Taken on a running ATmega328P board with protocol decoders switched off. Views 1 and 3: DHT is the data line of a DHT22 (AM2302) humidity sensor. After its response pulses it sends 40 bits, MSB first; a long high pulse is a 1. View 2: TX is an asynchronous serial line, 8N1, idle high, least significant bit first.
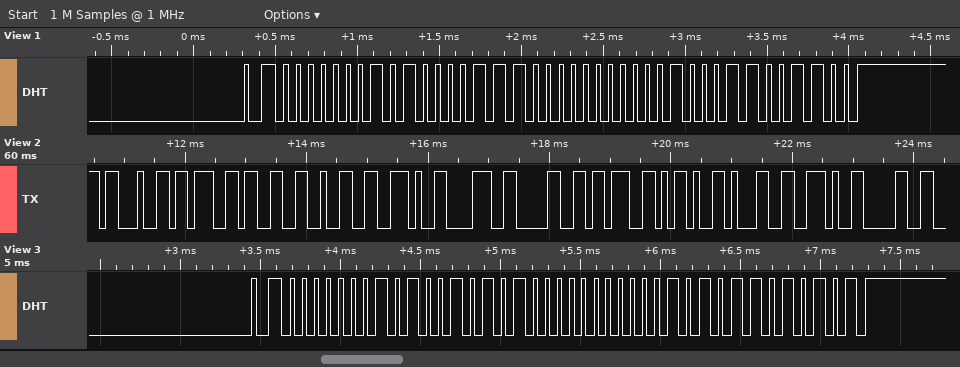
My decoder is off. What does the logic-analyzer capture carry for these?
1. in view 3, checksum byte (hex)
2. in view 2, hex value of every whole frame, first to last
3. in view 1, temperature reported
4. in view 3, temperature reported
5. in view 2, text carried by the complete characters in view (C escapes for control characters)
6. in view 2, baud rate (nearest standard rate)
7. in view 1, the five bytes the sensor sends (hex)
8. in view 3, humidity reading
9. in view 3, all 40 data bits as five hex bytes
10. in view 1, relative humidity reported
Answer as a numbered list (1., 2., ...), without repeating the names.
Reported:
1. 0xD5
2. 23 3B 33 32 2E 38 30 3B 2D 31 2E 30
3. -0.8 °C
4. -1.0 °C
5. "#;32.80;-1.0"
6. 9600 baud
7. 01 43 80 08 CC
8. 33.0 %
9. 01 4A 80 0A D5
10. 32.3 %
